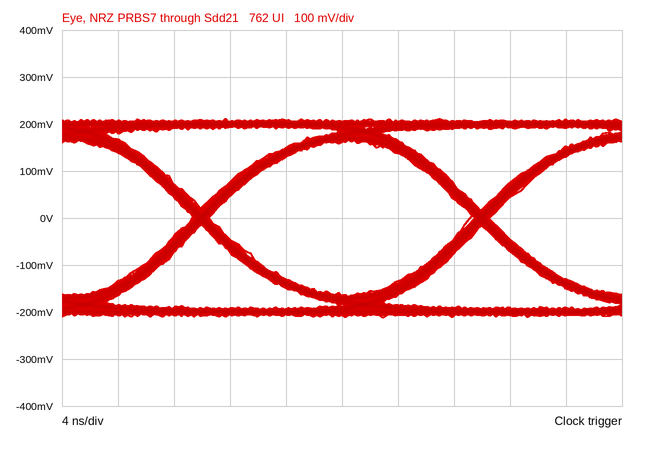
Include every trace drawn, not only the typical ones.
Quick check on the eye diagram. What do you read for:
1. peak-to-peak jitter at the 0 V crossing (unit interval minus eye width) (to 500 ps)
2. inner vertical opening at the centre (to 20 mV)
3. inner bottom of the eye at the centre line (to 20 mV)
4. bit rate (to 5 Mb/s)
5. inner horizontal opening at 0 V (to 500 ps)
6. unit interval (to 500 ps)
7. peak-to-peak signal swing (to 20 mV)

1.5 ns
320 mV
-160 mV
50 Mb/s
18.5 ns
20.0 ns
420 mV
